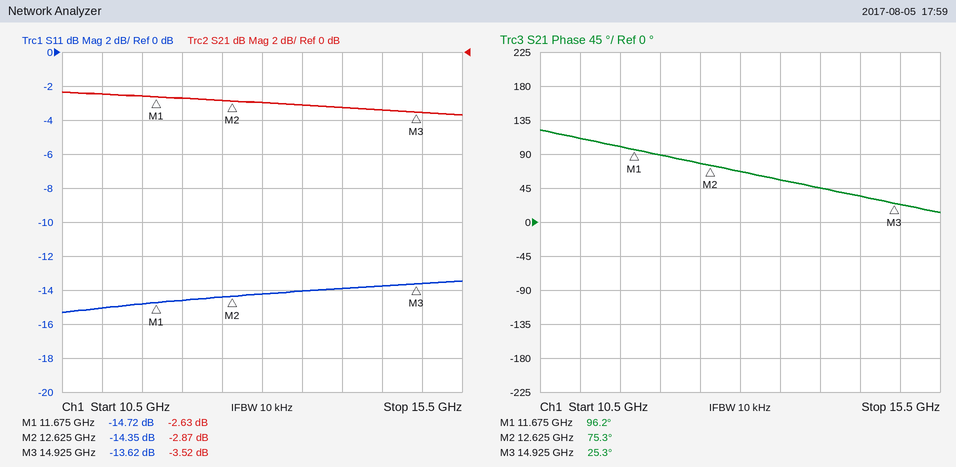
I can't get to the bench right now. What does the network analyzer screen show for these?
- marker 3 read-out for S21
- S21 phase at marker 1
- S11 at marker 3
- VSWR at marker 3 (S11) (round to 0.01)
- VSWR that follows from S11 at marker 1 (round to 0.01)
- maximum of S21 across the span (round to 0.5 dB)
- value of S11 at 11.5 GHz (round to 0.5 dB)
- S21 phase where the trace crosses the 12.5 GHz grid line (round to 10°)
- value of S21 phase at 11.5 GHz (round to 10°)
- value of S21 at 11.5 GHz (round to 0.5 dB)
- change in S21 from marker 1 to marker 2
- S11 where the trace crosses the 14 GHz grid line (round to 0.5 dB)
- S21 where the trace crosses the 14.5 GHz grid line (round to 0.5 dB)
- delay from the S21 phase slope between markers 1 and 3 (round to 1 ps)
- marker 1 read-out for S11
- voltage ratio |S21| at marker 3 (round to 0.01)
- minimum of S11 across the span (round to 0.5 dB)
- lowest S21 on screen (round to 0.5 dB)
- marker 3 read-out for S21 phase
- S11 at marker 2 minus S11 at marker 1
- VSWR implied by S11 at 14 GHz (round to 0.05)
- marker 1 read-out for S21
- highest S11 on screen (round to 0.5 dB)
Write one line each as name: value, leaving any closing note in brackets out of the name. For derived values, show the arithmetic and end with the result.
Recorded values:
marker 3 read-out for S21: -3.52 dB
S21 phase at marker 1: 96.2°
S11 at marker 3: -13.62 dB
VSWR at marker 3 (S11): (1 + 0.2084)/(1 − 0.2084) ≈ 1.53
VSWR that follows from S11 at marker 1: (1 + 0.1837)/(1 − 0.1837) ≈ 1.45
maximum of S21 across the span: -2.5 dB
value of S11 at 11.5 GHz: -15.0 dB
S21 phase where the trace crosses the 12.5 GHz grid line: 80°
value of S21 phase at 11.5 GHz: 100°
value of S21 at 11.5 GHz: -2.5 dB
change in S21 from marker 1 to marker 2: -2.87 − (-2.63) = -0.24 dB
S11 where the trace crosses the 14 GHz grid line: -14.0 dB
S21 where the trace crosses the 14.5 GHz grid line: -3.5 dB
delay from the S21 phase slope between markers 1 and 3: −(25.3° − (96.2°))/(360° × 3.25 GHz) ≈ 61 ps
marker 1 read-out for S11: -14.72 dB
voltage ratio |S21| at marker 3: 10^(-3.52/20) ≈ 0.67
minimum of S11 across the span: -15.5 dB
lowest S21 on screen: -3.5 dB
marker 3 read-out for S21 phase: 25.3°
S11 at marker 2 minus S11 at marker 1: -14.35 − (-14.72) = 0.37 dB
VSWR implied by S11 at 14 GHz: |Γ| = 10^(-14/20) = 0.1995; VSWR = (1 + 0.1995)/(1 − 0.1995) ≈ 1.50
marker 1 read-out for S21: -2.63 dB
highest S11 on screen: -13.5 dB
